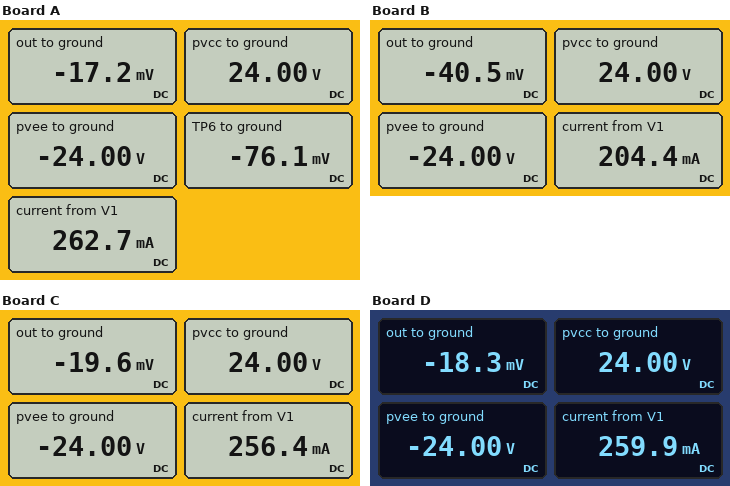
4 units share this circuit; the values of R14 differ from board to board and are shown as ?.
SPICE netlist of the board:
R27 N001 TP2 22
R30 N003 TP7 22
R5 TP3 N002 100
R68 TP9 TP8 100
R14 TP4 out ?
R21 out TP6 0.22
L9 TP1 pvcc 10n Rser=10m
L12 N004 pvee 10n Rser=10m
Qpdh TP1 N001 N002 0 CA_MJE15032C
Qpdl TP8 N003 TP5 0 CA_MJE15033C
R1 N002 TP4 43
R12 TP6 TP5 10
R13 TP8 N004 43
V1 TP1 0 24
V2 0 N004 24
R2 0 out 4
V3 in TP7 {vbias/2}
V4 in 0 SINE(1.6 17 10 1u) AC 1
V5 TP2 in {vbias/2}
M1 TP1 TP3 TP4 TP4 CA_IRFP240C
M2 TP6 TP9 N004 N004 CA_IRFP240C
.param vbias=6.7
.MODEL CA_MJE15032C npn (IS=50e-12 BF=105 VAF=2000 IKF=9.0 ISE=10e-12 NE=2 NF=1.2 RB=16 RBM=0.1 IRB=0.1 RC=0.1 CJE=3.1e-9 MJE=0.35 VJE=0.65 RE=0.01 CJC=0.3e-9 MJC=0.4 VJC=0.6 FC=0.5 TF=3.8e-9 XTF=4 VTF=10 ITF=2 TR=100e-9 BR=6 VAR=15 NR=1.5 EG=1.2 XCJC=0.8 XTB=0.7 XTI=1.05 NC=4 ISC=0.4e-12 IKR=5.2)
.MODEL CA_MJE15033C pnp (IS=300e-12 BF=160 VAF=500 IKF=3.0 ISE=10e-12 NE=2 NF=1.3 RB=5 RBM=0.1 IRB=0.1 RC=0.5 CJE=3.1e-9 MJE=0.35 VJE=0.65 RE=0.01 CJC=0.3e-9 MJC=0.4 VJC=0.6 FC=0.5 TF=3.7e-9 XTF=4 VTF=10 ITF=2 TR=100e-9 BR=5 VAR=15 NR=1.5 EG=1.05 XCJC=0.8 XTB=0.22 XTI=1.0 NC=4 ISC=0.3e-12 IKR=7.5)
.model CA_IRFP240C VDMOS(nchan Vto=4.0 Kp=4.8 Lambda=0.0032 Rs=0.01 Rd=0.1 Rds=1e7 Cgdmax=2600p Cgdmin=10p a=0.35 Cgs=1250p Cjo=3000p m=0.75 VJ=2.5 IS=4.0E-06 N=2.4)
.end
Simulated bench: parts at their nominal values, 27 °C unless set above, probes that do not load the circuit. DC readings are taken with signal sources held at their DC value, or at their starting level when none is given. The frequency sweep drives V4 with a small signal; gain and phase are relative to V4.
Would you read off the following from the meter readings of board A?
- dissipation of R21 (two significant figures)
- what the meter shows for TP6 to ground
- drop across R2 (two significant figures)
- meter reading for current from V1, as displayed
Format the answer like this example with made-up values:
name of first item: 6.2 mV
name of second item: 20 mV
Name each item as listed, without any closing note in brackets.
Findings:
dissipation of R21: 16 mW
what the meter shows for TP6 to ground: -76.1 mV
drop across R2: 17 mV
meter reading for current from V1, as displayed: 262.7 mA
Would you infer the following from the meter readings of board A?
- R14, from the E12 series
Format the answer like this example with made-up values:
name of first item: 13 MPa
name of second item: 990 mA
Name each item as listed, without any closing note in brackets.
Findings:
R14, from the E12 series: 0.068 Ω
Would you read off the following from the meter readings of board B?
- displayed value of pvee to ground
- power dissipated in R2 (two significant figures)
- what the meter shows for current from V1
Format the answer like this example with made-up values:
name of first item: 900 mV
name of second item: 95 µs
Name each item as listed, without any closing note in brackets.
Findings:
displayed value of pvee to ground: -24.00 V
power dissipated in R2: 410 µW
what the meter shows for current from V1: 204.4 mA
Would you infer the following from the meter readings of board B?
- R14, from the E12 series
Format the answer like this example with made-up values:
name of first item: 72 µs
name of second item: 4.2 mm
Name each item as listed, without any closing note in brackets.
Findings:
R14, from the E12 series: 0.47 Ω
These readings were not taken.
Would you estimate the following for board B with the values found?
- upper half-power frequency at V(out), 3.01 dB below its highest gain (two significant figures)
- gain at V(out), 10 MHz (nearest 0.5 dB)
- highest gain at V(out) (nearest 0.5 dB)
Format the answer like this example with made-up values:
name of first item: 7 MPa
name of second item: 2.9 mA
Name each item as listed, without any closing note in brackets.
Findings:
upper half-power frequency at V(out), 3.01 dB below its highest gain: 8.3 MHz
gain at V(out), 10 MHz: -5.5 dB
highest gain at V(out): 0 dB
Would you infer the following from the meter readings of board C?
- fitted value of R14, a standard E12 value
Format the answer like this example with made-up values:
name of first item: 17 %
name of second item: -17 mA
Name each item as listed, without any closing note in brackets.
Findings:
fitted value of R14, a standard E12 value: 0.1 Ω
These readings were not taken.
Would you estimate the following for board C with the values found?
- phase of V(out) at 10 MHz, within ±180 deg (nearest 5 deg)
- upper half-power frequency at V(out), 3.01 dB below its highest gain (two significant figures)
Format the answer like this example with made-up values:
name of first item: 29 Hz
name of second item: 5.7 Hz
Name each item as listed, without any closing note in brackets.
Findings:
phase of V(out) at 10 MHz, within ±180 deg: -105 deg
upper half-power frequency at V(out), 3.01 dB below its highest gain: 8.9 MHz
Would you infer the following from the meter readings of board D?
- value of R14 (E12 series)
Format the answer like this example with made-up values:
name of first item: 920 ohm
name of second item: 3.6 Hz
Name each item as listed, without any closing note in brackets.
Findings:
value of R14: 0.082 Ω
